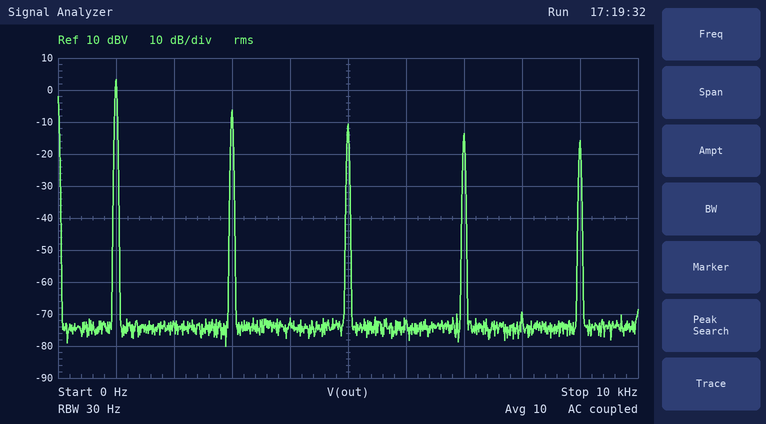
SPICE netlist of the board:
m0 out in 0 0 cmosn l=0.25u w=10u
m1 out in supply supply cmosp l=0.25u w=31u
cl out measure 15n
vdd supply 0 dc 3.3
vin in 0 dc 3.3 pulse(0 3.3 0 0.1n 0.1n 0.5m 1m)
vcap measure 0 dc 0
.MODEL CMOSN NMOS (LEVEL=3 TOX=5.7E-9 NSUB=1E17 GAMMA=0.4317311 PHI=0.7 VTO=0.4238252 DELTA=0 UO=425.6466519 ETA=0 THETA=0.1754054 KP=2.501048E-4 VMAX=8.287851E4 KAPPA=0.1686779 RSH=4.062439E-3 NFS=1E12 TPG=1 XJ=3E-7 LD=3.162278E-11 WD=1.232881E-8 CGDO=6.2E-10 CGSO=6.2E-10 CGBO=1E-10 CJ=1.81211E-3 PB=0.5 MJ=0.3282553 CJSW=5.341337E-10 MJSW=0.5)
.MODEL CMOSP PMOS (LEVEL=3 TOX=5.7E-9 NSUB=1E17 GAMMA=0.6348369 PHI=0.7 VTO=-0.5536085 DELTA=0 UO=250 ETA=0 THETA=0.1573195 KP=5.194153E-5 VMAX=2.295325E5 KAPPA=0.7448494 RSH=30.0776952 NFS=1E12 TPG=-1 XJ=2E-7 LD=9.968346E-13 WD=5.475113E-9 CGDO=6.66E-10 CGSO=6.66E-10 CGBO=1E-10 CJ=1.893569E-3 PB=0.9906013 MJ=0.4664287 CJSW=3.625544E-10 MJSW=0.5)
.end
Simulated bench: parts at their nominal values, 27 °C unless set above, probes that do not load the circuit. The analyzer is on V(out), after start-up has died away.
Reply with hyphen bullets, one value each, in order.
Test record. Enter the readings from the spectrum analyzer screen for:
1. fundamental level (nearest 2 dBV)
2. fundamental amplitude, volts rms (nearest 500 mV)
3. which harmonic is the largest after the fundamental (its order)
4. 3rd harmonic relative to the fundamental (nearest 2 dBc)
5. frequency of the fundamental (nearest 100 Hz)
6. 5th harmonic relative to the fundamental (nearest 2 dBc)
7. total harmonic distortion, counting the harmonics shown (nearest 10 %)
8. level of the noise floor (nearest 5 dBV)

- 4 dBV
- 1.5 V
- 3
- -10 dBc
- 1.0 kHz
- -14 dBc
- 40 %
- -75 dBV
